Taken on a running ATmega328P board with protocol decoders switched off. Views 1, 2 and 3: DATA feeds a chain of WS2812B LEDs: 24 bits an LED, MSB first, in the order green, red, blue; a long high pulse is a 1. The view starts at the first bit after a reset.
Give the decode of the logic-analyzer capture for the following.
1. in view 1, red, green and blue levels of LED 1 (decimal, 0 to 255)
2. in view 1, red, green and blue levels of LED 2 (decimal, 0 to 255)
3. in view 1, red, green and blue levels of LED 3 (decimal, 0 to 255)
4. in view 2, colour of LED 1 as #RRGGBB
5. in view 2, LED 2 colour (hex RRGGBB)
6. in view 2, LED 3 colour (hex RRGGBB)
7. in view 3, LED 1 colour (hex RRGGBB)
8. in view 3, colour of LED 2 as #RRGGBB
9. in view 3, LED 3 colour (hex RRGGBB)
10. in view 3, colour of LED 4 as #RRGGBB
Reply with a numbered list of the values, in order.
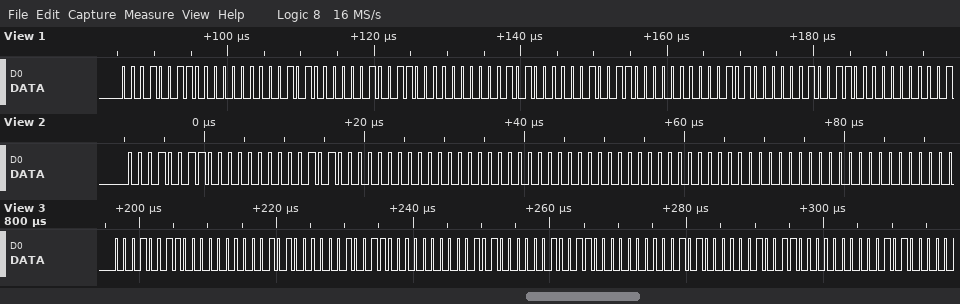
1. 0, 19, 40
2. 0, 19, 40
3. 0, 19, 40
4. #001328
5. #000000
6. #000000
7. #001328
8. #001328
9. #001328
10. #001328
